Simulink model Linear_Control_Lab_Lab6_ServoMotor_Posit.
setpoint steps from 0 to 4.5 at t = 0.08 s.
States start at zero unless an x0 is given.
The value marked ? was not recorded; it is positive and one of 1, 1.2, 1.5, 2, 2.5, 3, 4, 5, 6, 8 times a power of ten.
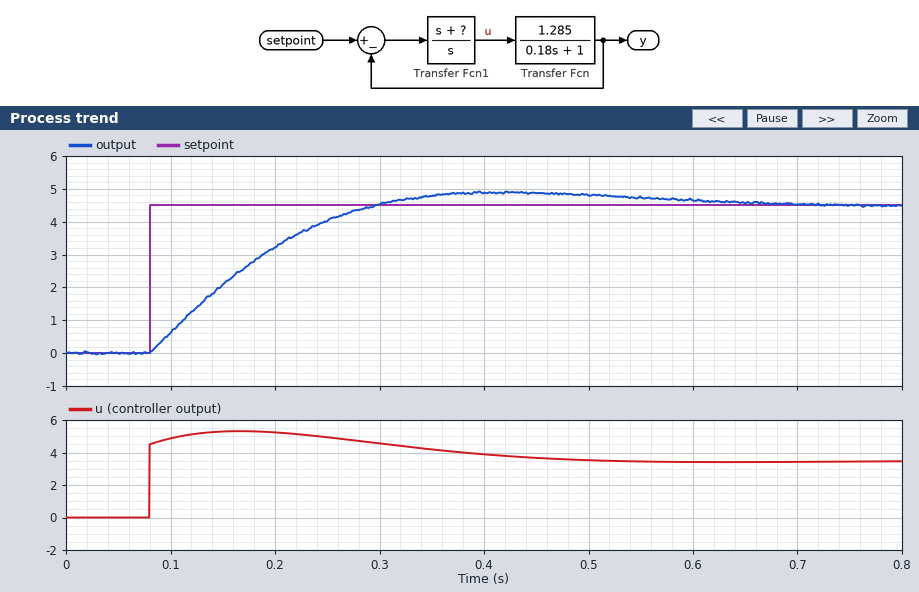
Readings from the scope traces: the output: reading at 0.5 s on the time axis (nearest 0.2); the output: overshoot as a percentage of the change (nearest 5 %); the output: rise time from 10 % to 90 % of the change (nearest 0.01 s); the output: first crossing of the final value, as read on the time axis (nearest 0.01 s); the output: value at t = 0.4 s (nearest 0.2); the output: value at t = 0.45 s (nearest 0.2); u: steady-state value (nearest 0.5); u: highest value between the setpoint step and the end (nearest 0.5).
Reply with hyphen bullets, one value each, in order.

- 4.8
- 10 %
- 0.16 s
- 0.30 s
- 4.8
- 4.8
- 3.5
- 5.5
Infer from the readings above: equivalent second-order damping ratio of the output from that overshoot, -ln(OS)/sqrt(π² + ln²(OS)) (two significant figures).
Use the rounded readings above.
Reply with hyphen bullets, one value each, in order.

- 0.59
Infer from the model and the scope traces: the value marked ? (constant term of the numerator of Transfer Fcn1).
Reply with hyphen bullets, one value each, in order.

- 12
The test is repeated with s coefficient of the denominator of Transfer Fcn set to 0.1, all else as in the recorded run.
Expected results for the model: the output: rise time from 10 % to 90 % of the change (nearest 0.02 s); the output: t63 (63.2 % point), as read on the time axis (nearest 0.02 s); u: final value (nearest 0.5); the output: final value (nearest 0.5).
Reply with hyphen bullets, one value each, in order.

- 0.14 s
- 0.16 s
- 3.5
- 4.5
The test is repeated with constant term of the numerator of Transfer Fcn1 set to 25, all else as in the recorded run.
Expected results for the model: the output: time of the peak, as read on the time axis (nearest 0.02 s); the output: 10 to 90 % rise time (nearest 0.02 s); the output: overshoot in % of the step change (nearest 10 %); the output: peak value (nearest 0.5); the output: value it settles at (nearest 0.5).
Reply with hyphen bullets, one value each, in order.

- 0.30 s
- 0.10 s
- 20 %
- 5.5
- 4.5
